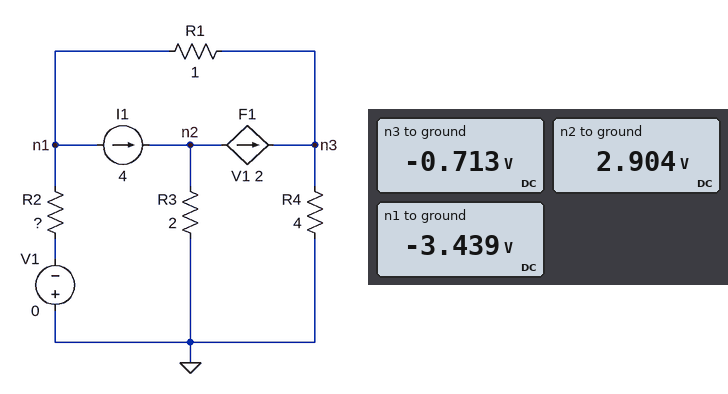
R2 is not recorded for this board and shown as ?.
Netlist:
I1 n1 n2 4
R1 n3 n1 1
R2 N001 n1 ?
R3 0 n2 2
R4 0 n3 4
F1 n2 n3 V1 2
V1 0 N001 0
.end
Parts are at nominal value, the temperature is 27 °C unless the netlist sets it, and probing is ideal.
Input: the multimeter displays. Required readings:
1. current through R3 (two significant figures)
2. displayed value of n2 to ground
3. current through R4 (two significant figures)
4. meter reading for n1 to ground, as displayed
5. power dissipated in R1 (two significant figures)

1.5 A
2.904 V
180 mA
-3.439 V
7.4 W
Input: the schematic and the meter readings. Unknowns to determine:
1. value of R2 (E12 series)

2.7 Ω
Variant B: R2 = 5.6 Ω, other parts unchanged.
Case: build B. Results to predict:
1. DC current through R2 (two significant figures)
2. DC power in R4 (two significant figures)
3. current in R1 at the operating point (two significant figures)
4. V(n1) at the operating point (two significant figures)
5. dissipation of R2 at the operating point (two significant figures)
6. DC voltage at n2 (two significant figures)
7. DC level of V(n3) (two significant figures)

1.1 A
2.4 W
2.9 A
-6.0 V
6.5 W
3.7 V
-3.1 V
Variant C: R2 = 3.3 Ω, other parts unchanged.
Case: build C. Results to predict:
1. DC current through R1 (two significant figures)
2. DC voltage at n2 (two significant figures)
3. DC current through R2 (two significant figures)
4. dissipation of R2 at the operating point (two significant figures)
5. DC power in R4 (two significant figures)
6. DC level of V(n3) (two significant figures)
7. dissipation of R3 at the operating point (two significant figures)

2.8 A
3.1 V
1.2 A
5.0 W
410 mW
-1.3 V
4.8 W
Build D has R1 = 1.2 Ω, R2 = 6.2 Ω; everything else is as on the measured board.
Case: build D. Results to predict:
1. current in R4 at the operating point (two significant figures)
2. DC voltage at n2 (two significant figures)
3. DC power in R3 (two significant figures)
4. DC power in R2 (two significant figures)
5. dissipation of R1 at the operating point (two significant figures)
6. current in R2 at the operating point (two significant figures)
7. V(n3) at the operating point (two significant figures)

780 mA
3.7 V
6.9 W
7.1 W
10 W
1.1 A
-3.1 V
